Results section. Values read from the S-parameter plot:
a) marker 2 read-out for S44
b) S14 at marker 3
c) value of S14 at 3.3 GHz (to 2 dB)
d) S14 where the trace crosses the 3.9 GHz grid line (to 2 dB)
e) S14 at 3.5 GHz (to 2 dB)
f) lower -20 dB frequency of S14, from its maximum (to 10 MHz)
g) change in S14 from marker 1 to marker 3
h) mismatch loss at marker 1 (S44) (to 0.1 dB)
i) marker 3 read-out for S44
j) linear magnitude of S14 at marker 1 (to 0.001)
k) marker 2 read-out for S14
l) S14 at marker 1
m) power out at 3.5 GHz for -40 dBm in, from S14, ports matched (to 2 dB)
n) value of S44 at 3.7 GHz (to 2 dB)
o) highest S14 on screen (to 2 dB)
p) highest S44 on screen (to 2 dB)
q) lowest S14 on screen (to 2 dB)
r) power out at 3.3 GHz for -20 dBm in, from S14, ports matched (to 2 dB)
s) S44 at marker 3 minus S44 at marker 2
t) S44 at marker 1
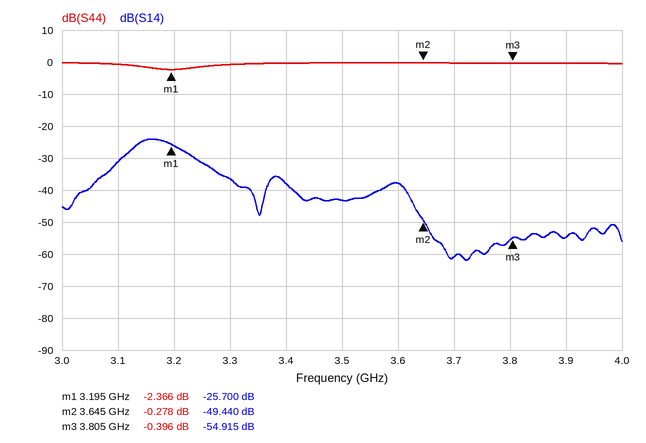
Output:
-0.278 dB
-54.915 dB
-36 dB
-54 dB
-44 dB
3.02 GHz
-29.215 dB
3.8 dB
-0.396 dB
0.052
-49.440 dB
-25.700 dB
-84 dBm
0 dB
-24 dB
0 dB
-62 dB
-56 dBm
-0.118 dB
-2.366 dB
